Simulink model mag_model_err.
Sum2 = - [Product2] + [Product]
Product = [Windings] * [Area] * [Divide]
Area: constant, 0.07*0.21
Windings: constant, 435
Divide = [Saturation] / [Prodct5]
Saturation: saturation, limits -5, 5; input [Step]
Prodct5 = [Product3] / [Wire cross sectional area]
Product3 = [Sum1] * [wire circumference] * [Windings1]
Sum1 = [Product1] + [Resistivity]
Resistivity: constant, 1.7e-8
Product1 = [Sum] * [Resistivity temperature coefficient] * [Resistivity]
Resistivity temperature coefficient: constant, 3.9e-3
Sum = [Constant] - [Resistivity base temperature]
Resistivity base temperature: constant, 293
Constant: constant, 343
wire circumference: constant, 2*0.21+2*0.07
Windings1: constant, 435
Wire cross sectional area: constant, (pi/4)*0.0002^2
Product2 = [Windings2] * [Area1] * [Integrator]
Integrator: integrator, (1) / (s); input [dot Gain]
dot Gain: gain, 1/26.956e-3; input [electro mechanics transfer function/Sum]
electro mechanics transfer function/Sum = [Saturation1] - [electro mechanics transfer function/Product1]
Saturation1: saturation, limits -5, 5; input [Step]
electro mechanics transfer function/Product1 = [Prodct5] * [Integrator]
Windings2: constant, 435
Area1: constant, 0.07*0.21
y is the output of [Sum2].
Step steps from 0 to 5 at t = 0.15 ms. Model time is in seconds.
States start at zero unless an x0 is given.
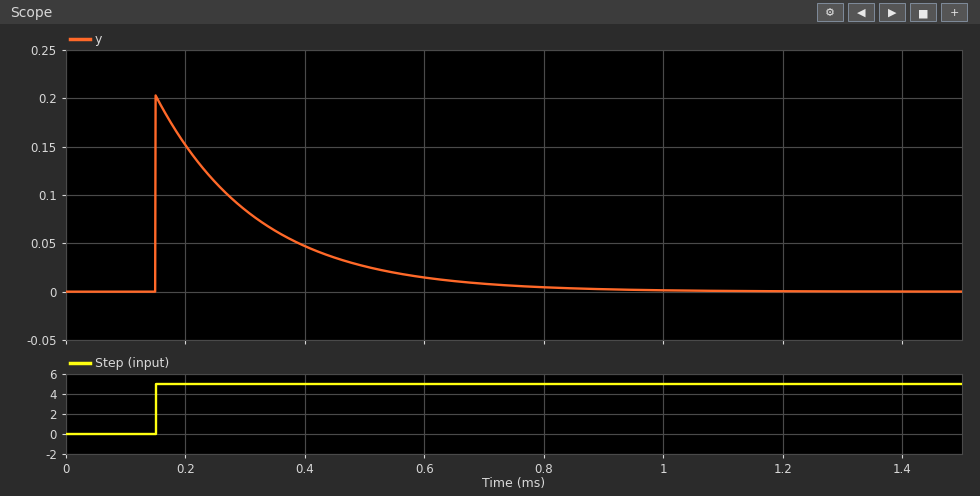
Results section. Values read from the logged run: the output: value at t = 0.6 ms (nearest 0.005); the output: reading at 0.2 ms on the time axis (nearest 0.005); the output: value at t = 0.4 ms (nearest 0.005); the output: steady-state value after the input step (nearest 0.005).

0.015
0.150
0.045
0.000
